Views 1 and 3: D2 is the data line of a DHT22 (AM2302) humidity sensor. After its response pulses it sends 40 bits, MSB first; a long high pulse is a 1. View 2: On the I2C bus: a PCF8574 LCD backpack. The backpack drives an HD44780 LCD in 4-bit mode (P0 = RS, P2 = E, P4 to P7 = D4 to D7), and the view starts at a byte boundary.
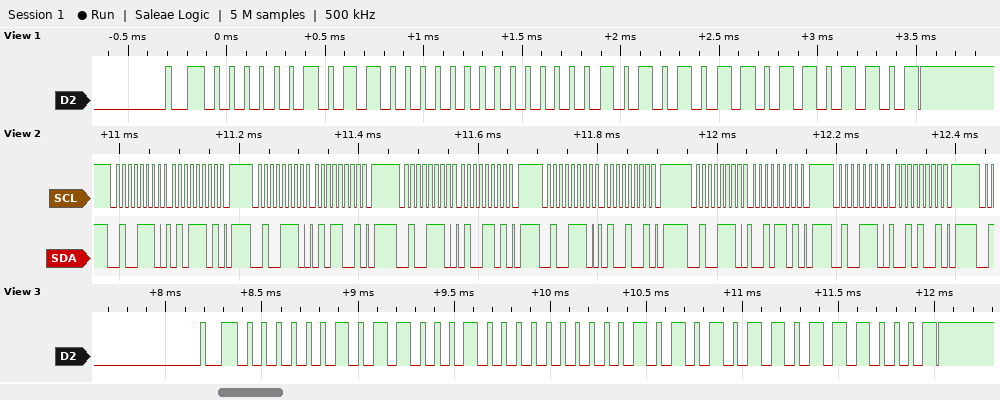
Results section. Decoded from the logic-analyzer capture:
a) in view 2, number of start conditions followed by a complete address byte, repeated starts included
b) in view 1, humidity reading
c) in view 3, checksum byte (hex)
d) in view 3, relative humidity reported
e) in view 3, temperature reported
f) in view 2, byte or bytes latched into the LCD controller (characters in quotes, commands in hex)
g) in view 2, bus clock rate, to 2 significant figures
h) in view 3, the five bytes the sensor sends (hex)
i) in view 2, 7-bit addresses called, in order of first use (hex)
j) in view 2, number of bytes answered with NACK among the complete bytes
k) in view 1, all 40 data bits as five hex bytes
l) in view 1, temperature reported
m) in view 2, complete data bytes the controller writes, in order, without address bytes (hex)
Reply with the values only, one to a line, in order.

6
70.4 %
0x71
70.8 %
17.1 °C
'T'
100 kHz
02 C4 00 AB 71
0x27
0
02 C0 00 AB 6D
17.1 °C
5D 59 4D 49 2D 29
